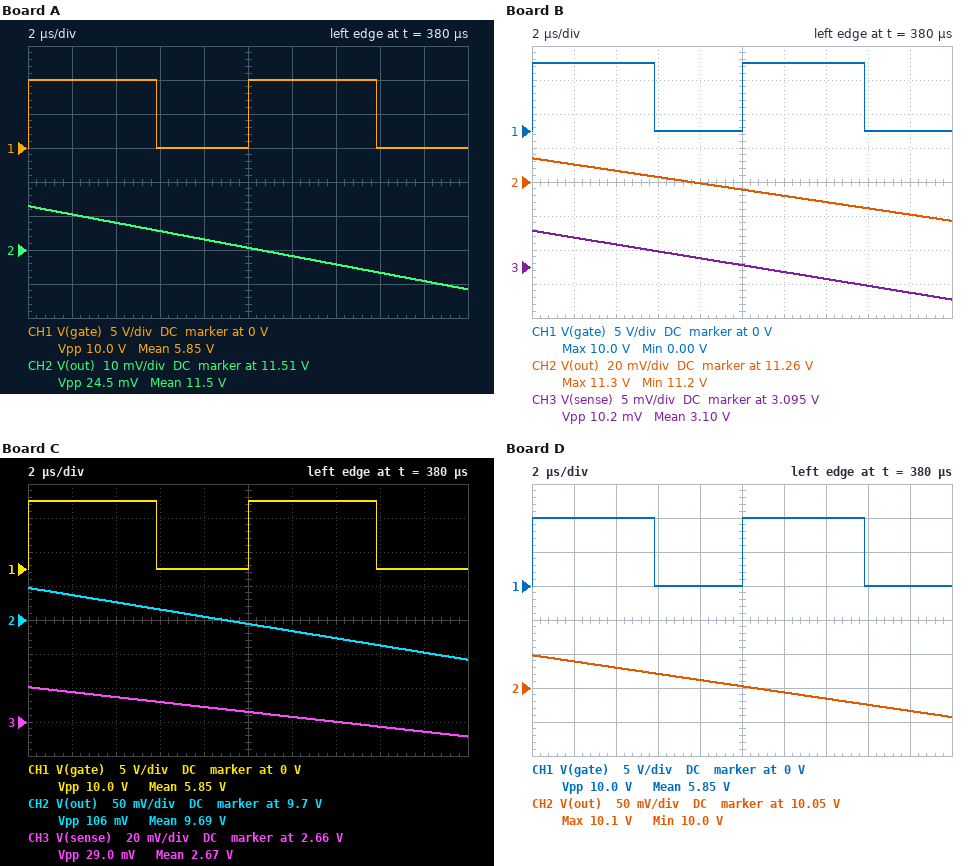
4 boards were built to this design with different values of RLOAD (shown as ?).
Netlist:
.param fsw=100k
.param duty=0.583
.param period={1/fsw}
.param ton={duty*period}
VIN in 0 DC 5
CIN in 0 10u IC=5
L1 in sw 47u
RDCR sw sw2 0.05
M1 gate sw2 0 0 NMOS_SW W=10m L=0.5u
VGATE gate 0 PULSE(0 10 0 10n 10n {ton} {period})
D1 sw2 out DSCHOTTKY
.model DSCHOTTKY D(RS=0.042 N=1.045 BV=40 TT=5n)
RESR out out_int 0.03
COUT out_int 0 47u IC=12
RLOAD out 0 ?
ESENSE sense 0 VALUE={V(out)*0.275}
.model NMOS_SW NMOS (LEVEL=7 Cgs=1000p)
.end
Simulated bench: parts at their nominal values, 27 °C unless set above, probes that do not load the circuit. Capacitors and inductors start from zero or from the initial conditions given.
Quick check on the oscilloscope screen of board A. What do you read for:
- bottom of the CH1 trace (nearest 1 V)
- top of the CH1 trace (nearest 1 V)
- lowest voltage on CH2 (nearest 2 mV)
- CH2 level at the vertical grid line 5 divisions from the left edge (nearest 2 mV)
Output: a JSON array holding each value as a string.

["0 V", "10 V", "11.498 V", "11.510 V"]
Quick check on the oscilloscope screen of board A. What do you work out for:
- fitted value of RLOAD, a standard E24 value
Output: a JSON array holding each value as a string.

["200 Ω"]
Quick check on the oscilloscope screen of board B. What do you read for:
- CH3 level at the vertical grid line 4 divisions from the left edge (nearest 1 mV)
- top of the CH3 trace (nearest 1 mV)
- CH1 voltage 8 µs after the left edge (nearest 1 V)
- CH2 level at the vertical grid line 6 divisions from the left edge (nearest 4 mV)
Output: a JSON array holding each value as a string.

["3.096 V", "3.100 V", "0 V", "11.252 V"]
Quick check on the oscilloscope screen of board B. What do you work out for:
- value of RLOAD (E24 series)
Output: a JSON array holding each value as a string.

["130 Ω"]
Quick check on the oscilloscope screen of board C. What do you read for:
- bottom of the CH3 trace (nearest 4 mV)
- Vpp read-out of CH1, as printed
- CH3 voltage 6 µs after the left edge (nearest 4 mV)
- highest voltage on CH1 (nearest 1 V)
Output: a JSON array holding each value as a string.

["2.652 V", "10.0 V", "2.672 V", "10 V"]
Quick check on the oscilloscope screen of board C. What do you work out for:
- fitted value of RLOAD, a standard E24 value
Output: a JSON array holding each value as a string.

["39 Ω"]
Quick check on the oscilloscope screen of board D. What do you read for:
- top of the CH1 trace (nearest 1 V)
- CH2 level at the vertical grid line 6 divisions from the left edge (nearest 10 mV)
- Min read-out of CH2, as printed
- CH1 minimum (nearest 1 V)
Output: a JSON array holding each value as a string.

["10 V", "10.04 V", "10.0 V", "0 V"]
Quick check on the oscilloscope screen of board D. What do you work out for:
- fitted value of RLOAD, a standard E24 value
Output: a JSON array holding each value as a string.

["47 Ω"]
